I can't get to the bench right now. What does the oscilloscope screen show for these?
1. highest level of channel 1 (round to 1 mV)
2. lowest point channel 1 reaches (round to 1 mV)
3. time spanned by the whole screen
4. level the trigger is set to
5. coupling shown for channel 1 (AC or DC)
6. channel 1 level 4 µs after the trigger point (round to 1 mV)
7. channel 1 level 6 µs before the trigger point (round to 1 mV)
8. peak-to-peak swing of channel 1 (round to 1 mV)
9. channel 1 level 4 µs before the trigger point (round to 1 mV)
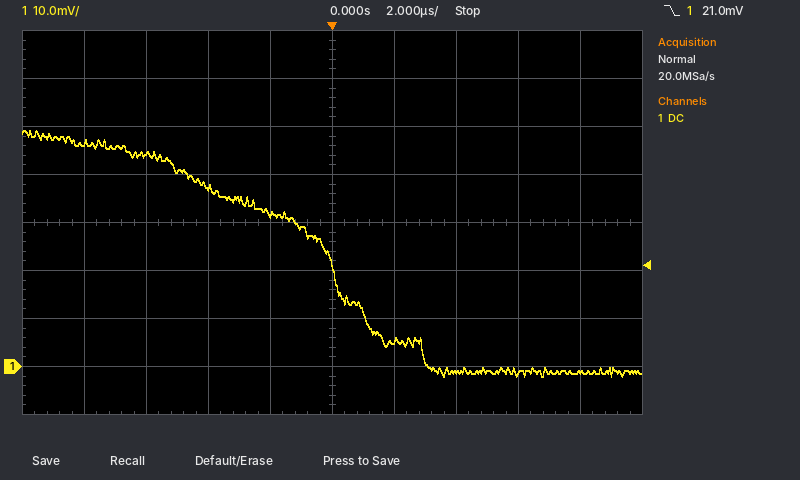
49 mV
-2 mV
20 µs
21.0 mV
DC
-1 mV
44 mV
51 mV
37 mV
